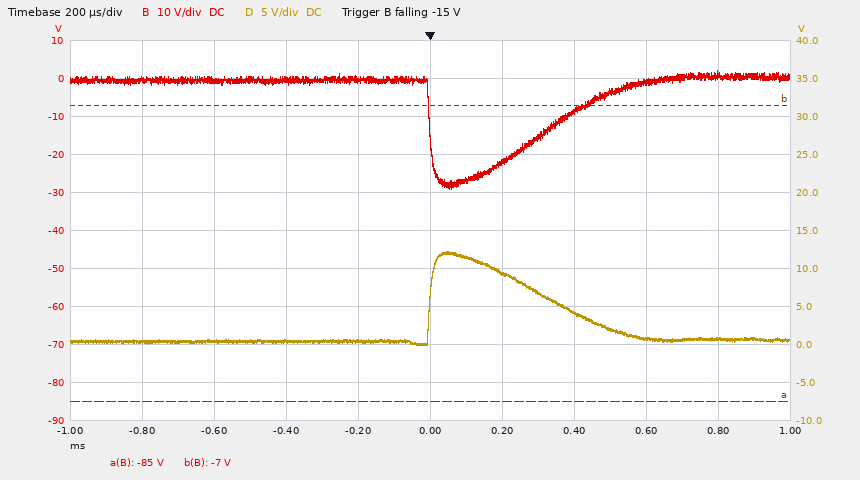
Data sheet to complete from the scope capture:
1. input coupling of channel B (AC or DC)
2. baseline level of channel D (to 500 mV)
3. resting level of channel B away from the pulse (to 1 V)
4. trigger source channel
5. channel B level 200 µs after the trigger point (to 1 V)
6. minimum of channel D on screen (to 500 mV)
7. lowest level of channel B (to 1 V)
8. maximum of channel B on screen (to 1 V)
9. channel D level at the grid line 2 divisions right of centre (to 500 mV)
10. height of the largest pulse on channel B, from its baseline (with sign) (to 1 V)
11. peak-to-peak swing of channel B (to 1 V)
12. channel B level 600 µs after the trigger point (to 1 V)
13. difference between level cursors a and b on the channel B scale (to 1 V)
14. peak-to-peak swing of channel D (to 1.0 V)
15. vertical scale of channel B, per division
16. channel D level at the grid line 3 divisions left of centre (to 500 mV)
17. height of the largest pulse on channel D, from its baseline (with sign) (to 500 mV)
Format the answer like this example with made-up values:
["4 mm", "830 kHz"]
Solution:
["DC", "500 mV", "0 V", "channel B", "-22 V", "0.0 V", "-29 V", "2 V", "4.0 V", "-29 V", "31 V", "-1 V", "78 V", "12.0 V", "10 V", "500 mV", "+12.0 V"]
